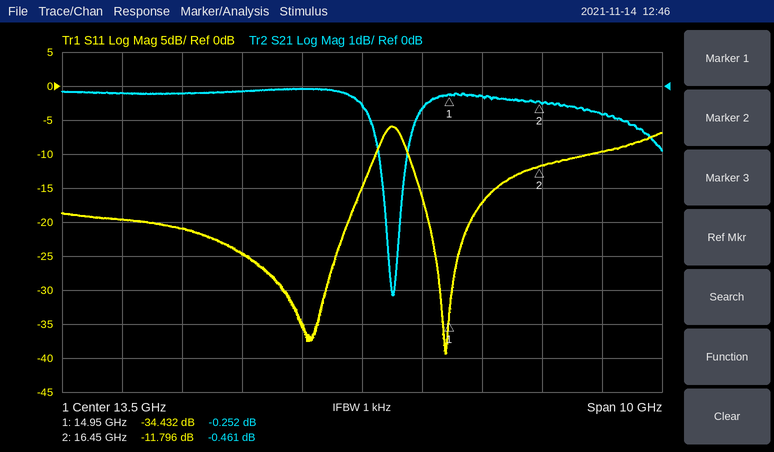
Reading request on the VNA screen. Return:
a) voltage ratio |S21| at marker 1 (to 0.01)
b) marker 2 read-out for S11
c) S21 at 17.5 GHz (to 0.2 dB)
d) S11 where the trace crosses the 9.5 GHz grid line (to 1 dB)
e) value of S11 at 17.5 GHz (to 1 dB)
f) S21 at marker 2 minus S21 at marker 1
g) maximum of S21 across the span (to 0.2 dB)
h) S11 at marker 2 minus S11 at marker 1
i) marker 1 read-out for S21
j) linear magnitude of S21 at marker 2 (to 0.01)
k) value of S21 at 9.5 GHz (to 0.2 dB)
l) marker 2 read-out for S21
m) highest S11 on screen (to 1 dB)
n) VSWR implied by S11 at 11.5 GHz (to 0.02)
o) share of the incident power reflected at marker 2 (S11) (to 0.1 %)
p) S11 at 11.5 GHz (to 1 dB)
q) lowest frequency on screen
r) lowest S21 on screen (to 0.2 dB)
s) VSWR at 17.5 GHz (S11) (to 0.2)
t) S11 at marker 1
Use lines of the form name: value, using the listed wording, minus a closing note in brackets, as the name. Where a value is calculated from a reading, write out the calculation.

voltage ratio |S21| at marker 1: 10^(-0.252/20) ≈ 0.97
marker 2 read-out for S11: -11.796 dB
S21 at 17.5 GHz: -0.8 dB
S11 where the trace crosses the 9.5 GHz grid line: -20 dB
value of S11 at 17.5 GHz: -10 dB
S21 at marker 2 minus S21 at marker 1: -0.461 − (-0.252) = -0.209 dB
maximum of S21 across the span: 0.0 dB
S11 at marker 2 minus S11 at marker 1: -11.796 − (-34.432) = 22.636 dB
marker 1 read-out for S21: -0.252 dB
linear magnitude of S21 at marker 2: 10^(-0.461/20) ≈ 0.95
value of S21 at 9.5 GHz: -0.2 dB
marker 2 read-out for S21: -0.461 dB
highest S11 on screen: -6 dB
VSWR implied by S11 at 11.5 GHz: |Γ| = 10^(-25/20) = 0.0562; VSWR = (1 + 0.0562)/(1 − 0.0562) ≈ 1.12
share of the incident power reflected at marker 2 (S11): 10^(-11.796/10) ≈ 6.6 %
S11 at 11.5 GHz: -25 dB
lowest frequency on screen: 8.5 GHz
lowest S21 on screen: -6.2 dB
VSWR at 17.5 GHz (S11): |Γ| = 10^(-10/20) = 0.3162; VSWR = (1 + 0.3162)/(1 − 0.3162) ≈ 1.92, so 2.0 to the nearest 0.2
S11 at marker 1: -34.432 dB
